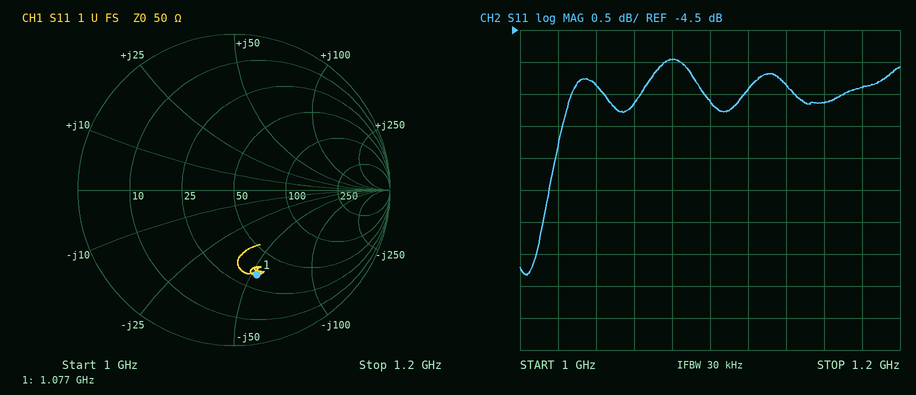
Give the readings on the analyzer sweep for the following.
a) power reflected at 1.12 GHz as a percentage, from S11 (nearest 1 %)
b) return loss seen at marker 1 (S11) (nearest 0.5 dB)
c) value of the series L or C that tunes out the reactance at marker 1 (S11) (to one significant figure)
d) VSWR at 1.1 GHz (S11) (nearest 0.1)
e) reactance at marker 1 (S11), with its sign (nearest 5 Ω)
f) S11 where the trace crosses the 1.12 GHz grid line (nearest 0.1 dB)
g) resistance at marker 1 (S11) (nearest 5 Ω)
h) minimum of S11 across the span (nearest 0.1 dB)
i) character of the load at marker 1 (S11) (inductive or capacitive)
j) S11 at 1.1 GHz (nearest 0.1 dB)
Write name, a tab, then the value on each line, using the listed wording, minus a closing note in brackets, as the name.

power reflected at 1.12 GHz as a percentage, from S11	29 %
return loss seen at marker 1 (S11)	5.0 dB
value of the series L or C that tunes out the reactance at marker 1 (S11)	8 nH
VSWR at 1.1 GHz (S11)	3.2
reactance at marker 1 (S11), with its sign	-55 Ω
S11 where the trace crosses the 1.12 GHz grid line	-5.4 dB
resistance at marker 1 (S11)	35 Ω
minimum of S11 across the span	-8.3 dB
character of the load at marker 1 (S11)	capacitive
S11 at 1.1 GHz	-5.6 dB
